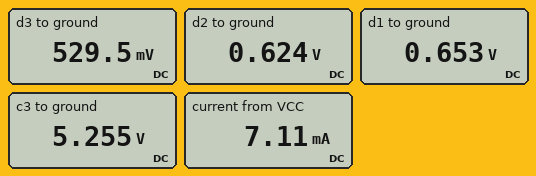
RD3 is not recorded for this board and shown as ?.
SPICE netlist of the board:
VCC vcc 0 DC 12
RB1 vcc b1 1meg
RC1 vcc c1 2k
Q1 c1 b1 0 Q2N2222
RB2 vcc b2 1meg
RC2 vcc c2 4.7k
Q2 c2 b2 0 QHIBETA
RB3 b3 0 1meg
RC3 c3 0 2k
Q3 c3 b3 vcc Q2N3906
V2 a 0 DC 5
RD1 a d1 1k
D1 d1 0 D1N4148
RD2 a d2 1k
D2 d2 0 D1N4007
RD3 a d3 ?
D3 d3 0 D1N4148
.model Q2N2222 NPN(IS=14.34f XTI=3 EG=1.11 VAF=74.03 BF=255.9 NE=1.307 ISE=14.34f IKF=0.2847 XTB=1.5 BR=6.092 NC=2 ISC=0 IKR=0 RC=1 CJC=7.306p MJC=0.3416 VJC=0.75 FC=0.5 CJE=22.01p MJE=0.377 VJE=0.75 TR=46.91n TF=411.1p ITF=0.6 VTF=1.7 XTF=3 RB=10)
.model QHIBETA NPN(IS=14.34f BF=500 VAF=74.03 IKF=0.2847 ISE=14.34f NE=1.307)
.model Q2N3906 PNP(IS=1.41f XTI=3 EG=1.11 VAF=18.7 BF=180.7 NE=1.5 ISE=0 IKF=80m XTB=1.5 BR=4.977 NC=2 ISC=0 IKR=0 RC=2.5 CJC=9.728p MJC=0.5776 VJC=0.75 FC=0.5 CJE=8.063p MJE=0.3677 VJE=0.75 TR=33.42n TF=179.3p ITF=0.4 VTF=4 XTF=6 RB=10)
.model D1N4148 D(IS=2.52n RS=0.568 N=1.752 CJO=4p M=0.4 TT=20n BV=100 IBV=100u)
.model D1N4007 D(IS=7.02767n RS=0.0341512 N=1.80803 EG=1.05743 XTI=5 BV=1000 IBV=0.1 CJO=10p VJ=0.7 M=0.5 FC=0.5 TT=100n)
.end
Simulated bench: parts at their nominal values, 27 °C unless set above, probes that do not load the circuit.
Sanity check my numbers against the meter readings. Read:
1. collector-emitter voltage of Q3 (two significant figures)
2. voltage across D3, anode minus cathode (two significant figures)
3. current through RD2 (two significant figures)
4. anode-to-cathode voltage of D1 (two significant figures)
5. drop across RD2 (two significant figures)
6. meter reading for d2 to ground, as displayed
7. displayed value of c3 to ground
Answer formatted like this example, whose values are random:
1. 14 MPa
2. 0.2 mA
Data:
1. -6.7 V
2. 530 mV
3. 4.4 mA
4. 650 mV
5. 4.4 V
6. 0.624 V
7. 5.255 V
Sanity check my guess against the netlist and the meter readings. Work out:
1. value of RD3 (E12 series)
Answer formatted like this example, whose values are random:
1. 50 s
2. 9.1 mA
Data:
1. 15 kΩ
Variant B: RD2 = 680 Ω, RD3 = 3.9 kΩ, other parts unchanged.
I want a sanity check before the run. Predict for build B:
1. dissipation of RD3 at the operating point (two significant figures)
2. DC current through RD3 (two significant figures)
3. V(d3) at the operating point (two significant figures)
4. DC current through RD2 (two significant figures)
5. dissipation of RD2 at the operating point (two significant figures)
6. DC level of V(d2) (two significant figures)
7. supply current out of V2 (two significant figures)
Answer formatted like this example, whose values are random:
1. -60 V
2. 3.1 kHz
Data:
1. 5.0 mW
2. 1.1 mA
3. 590 mV
4. 6.4 mA
5. 28 mW
6. 640 mV
7. 12 mA
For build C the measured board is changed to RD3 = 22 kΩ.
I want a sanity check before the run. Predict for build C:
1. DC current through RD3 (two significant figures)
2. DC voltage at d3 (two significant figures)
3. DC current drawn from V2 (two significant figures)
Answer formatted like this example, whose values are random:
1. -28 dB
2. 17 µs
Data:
1. 200 µA
2. 510 mV
3. 8.9 mA
